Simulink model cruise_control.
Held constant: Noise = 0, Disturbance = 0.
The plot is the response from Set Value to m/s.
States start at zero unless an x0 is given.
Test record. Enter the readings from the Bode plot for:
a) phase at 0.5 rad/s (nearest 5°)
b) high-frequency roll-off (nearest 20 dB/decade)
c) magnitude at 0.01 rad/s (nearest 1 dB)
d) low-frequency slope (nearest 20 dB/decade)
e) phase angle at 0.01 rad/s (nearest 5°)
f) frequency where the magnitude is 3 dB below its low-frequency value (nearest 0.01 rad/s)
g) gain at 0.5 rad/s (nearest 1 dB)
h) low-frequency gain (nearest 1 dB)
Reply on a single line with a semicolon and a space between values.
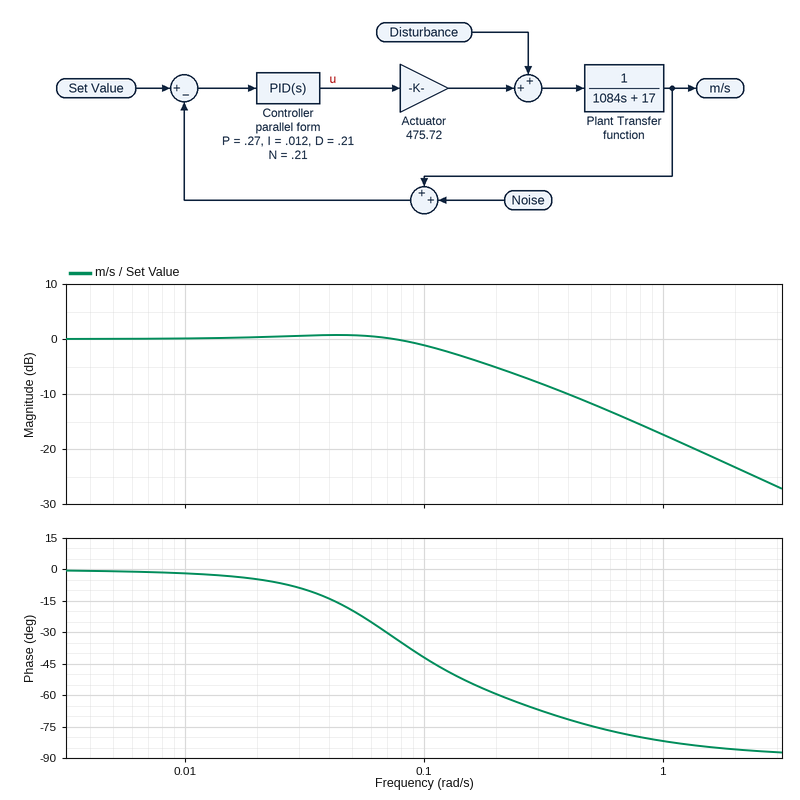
-75°; -20 dB/decade; 0 dB; 0 dB/decade; 0°; 0.14 rad/s; -12 dB; 0 dB
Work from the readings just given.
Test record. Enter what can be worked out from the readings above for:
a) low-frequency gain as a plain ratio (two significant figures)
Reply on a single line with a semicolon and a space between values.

1.0
